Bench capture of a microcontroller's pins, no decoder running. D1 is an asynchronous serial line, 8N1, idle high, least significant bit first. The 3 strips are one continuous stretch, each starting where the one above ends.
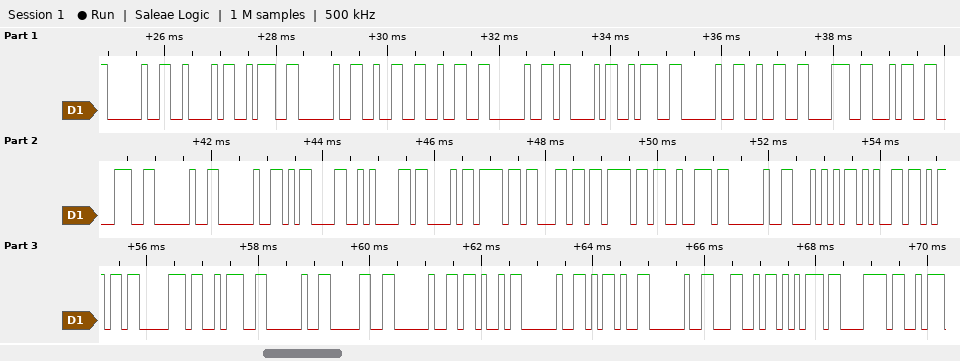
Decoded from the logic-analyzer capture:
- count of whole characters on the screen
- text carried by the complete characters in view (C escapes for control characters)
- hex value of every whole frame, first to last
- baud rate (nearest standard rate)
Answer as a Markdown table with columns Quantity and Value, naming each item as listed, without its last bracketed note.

| Quantity | Value |
|---|---|
| count of whole characters on the screen | 39 |
| text carried by the complete characters in view | " B: 22 C: 2848  \r\nColor Temp: 0 K - Lux" |
| hex value of every whole frame, first to last | 20 42 3A 20 32 32 20 43 3A 20 32 38 34 38 20 20 0D 0A 43 6F 6C 6F 72 20 54 65 6D 70 3A 20 30 20 4B 20 2D 20 4C 75 78 |
| baud rate | 9600 baud |
